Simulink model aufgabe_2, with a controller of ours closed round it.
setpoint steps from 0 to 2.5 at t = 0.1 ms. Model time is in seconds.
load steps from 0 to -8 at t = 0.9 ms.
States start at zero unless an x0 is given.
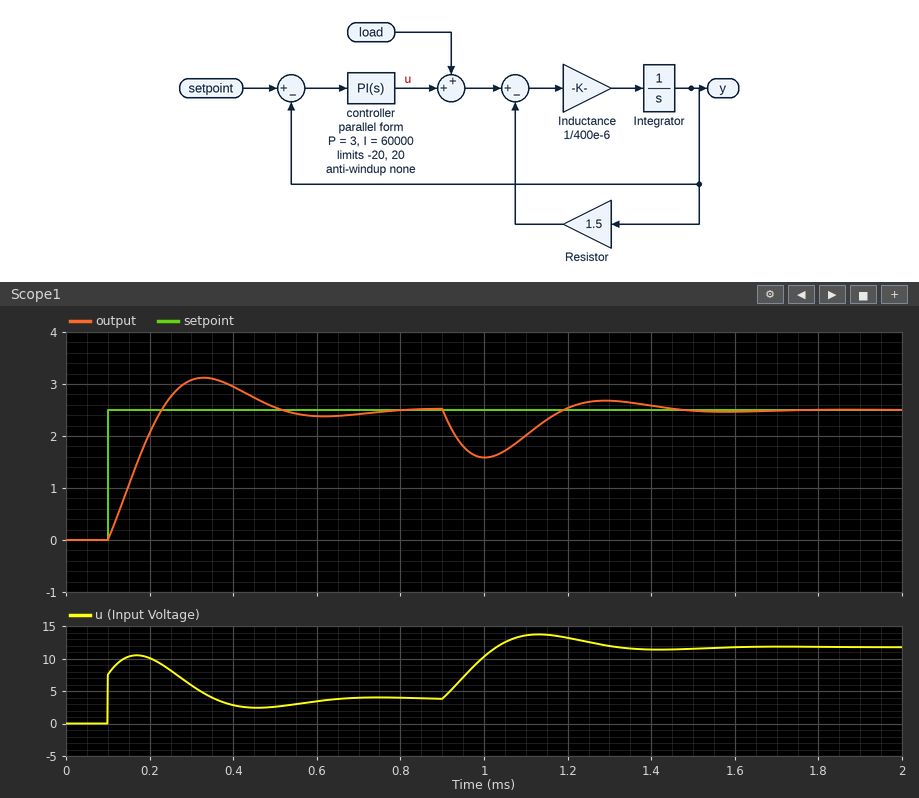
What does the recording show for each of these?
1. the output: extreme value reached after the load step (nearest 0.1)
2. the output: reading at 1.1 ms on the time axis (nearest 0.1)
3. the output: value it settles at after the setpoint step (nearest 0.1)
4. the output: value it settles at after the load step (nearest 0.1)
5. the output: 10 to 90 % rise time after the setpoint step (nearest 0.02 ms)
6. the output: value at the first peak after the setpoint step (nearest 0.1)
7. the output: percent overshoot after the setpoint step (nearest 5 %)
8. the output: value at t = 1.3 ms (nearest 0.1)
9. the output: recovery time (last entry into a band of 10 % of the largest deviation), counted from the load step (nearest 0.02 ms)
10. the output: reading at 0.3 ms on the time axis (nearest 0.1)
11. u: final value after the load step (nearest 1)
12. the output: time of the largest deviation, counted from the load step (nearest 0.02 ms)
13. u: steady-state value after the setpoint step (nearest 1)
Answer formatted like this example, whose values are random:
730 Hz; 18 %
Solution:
1.6; 2.0; 2.5; 2.5; 0.10 ms; 3.1; 25 %; 2.7; 0.50 ms; 3.1; 12; 0.10 ms; 4
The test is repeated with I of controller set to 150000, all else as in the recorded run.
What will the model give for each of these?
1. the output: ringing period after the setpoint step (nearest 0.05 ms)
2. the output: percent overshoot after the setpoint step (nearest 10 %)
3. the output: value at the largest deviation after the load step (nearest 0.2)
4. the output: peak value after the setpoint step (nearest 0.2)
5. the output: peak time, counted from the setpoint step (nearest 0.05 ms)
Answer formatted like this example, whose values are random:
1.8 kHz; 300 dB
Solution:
0.35 ms; 40 %; 1.8; 3.6; 0.15 ms
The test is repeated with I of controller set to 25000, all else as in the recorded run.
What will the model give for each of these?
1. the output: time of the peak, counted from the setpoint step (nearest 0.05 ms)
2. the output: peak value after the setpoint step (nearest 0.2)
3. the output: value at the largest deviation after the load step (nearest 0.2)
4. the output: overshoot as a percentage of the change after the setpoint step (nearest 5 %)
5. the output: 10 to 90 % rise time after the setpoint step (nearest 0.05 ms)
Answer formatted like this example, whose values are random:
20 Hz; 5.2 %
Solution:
0.35 ms; 2.8; 1.4; 10 %; 0.15 ms
